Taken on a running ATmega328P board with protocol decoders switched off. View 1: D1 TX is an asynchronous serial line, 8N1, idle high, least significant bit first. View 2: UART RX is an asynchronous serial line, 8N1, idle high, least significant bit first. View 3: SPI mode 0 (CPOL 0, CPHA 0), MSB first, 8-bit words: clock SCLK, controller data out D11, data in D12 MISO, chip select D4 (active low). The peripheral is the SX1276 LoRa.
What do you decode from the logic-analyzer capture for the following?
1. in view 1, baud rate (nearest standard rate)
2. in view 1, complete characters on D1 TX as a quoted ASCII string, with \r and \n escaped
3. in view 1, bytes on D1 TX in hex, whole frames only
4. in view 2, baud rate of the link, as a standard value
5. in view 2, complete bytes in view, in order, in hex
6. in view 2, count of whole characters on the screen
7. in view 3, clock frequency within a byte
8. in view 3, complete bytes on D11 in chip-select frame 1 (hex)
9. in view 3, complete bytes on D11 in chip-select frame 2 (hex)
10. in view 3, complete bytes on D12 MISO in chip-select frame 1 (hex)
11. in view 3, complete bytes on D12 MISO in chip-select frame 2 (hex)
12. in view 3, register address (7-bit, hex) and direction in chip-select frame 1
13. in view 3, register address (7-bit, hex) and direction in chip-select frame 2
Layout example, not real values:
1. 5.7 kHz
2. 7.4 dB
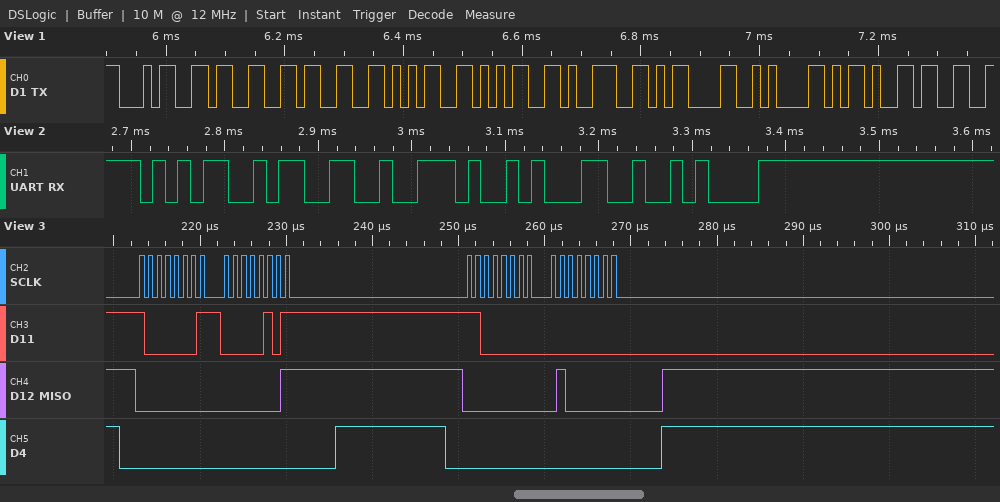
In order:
1. 74880 baud
2. "433559\r\n-3"
3. 0x34 0x33 0x33 0x35 0x35 0x39 0x0D 0x0A 0x2D 0x33
4. 74880 baud
5. 35 33 2E 31 0A
6. 5
7. 1 MHz
8. 81 05
9. C0 00
10. 00 01
11. 00 40
12. 0x01 write
13. 0x40 write
